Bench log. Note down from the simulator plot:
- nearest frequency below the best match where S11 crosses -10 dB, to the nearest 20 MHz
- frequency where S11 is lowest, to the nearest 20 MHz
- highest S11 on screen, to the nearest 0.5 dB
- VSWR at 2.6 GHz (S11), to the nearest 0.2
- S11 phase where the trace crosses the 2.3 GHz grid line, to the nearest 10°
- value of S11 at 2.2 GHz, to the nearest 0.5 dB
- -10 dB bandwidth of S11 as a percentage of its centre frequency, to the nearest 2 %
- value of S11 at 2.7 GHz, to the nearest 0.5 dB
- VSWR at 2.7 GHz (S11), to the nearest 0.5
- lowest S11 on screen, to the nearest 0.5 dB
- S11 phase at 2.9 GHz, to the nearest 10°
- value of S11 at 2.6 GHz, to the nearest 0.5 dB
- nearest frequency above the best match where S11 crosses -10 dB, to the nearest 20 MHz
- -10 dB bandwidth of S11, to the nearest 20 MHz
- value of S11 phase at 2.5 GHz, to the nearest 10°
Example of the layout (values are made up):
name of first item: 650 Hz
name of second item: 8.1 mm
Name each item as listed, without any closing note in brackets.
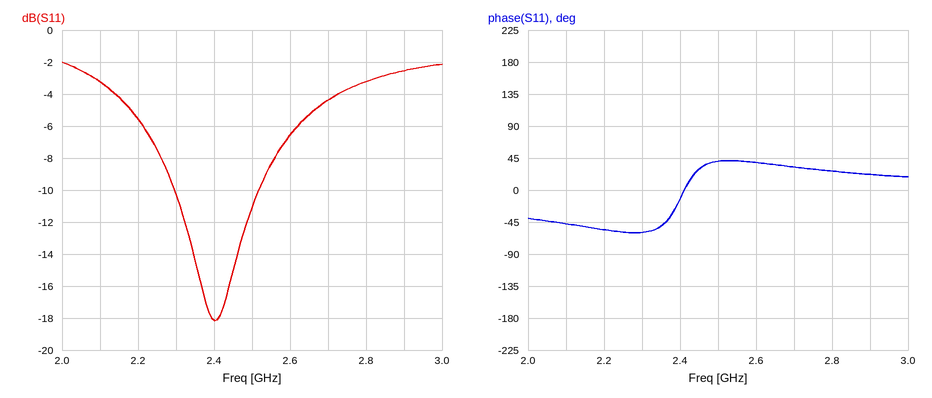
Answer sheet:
nearest frequency below the best match where S11 crosses -10 dB, to the nearest 20 MHz: 2.30 GHz
frequency where S11 is lowest, to the nearest 20 MHz: 2.40 GHz
highest S11 on screen, to the nearest 0.5 dB: -2.0 dB
VSWR at 2.6 GHz (S11), to the nearest 0.2: 2.8
S11 phase where the trace crosses the 2.3 GHz grid line, to the nearest 10°: -60°
value of S11 at 2.2 GHz, to the nearest 0.5 dB: -5.5 dB
-10 dB bandwidth of S11 as a percentage of its centre frequency, to the nearest 2 %: 10 %
value of S11 at 2.7 GHz, to the nearest 0.5 dB: -4.5 dB
VSWR at 2.7 GHz (S11), to the nearest 0.5: 4.0
lowest S11 on screen, to the nearest 0.5 dB: -18.0 dB
S11 phase at 2.9 GHz, to the nearest 10°: 20°
value of S11 at 2.6 GHz, to the nearest 0.5 dB: -6.5 dB
nearest frequency above the best match where S11 crosses -10 dB, to the nearest 20 MHz: 2.52 GHz
-10 dB bandwidth of S11, to the nearest 20 MHz: 220 MHz
value of S11 phase at 2.5 GHz, to the nearest 10°: 40°
